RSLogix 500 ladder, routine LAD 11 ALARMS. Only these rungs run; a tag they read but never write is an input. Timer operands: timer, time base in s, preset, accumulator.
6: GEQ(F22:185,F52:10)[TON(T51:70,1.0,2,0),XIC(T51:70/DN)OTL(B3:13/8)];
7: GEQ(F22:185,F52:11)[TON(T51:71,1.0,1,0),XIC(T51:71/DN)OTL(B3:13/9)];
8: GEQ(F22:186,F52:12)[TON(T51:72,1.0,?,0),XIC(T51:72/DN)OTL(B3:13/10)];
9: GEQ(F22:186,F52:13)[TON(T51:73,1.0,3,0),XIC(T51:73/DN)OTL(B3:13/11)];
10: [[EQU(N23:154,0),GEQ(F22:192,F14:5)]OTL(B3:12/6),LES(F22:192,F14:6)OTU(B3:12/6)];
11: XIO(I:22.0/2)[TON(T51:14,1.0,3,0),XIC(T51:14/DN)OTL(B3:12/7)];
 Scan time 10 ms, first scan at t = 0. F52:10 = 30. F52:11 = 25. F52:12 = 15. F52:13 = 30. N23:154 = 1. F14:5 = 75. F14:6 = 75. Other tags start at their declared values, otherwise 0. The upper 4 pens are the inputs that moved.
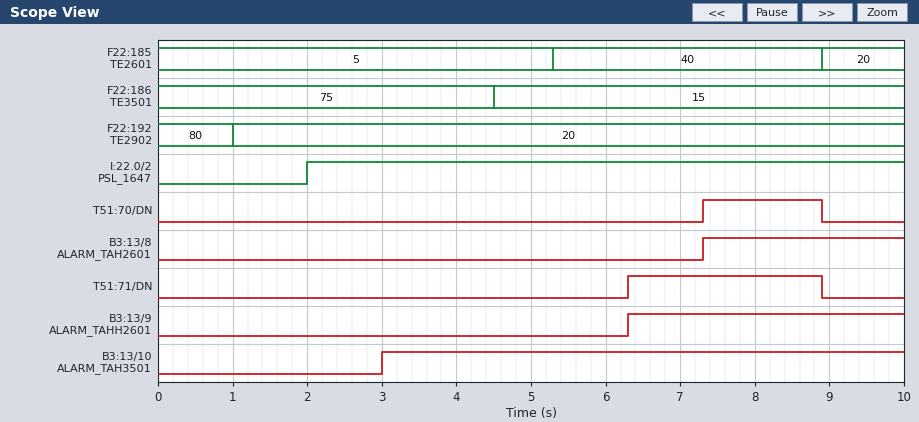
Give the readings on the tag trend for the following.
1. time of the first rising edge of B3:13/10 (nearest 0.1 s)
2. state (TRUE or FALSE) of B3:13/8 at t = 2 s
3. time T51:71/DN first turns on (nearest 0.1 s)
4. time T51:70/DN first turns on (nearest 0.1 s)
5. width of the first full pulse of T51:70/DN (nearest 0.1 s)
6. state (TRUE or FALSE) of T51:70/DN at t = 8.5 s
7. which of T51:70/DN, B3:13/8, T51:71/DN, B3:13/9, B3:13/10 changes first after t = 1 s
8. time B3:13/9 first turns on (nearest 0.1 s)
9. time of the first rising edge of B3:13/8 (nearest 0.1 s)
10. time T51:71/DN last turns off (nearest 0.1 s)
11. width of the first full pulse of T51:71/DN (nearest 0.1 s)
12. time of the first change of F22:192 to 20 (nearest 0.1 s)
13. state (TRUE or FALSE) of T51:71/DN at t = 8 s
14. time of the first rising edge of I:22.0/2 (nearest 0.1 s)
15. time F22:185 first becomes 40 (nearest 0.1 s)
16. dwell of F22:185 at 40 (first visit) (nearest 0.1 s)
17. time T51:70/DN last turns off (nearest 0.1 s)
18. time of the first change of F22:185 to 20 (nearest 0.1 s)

3.0 s
FALSE
6.3 s
7.3 s
1.6 s
TRUE
B3:13/10
6.3 s
7.3 s
8.9 s
2.6 s
1.0 s
TRUE
2.0 s
5.3 s
3.6 s
8.9 s
8.9 s
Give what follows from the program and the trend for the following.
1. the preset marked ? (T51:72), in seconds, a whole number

3 s
